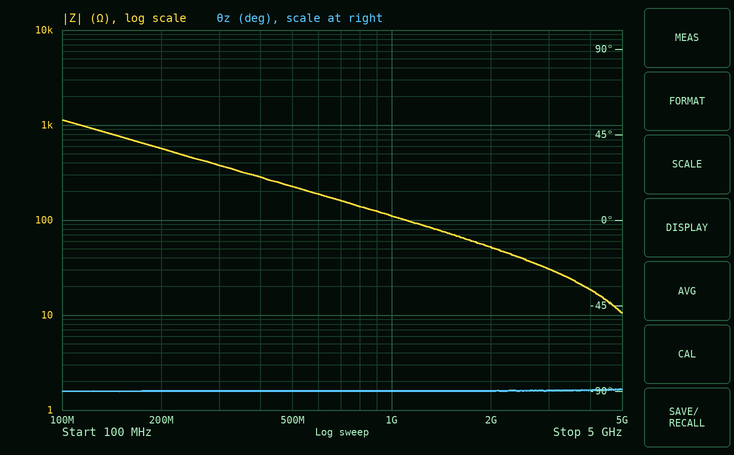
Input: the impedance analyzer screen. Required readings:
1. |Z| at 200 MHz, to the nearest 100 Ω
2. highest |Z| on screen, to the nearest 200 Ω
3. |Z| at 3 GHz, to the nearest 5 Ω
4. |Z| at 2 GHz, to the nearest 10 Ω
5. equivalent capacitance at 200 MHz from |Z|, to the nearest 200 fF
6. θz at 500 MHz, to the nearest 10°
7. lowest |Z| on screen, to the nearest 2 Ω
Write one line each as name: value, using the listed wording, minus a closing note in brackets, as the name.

|Z| at 200 MHz, to the nearest 100 Ω: 600 Ω
highest |Z| on screen, to the nearest 200 Ω: 1.2 kΩ
|Z| at 3 GHz, to the nearest 5 Ω: 30 Ω
|Z| at 2 GHz, to the nearest 10 Ω: 50 Ω
equivalent capacitance at 200 MHz from |Z|, to the nearest 200 fF: 1.4 pF
θz at 500 MHz, to the nearest 10°: -90°
lowest |Z| on screen, to the nearest 2 Ω: 10 Ω
